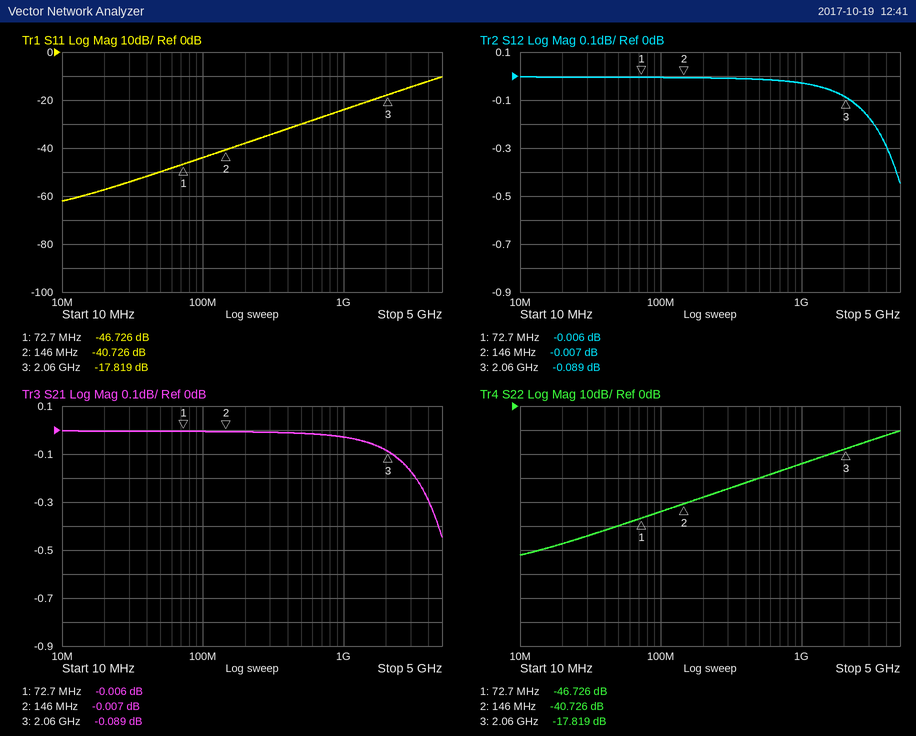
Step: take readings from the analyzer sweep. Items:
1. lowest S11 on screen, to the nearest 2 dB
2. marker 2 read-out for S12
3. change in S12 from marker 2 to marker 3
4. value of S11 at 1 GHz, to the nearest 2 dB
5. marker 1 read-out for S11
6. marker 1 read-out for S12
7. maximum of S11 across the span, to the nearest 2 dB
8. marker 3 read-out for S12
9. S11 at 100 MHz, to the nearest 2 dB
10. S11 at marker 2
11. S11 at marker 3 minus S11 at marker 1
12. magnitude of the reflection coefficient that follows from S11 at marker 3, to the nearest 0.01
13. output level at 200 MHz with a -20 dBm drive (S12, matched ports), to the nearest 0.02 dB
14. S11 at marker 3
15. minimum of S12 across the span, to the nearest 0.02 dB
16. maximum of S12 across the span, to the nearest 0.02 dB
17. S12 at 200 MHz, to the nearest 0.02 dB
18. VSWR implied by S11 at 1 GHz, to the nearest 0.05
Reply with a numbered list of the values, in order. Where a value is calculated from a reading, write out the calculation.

1. -62 dB
2. -0.007 dB
3. -0.089 − (-0.007) = -0.082 dB
4. -24 dB
5. -46.726 dB
6. -0.006 dB
7. -10 dB
8. -0.089 dB
9. -44 dB
10. -40.726 dB
11. -17.819 − (-46.726) = 28.907 dB
12. 10^(-17.819/20) ≈ 0.13
13. -20 dBm + (0.00 dB) = -20.00 dBm
14. -17.819 dB
15. -0.44 dB
16. 0.00 dB
17. 0.00 dB
18. |Γ| = 10^(-24/20) = 0.0631; VSWR = (1 + 0.0631)/(1 − 0.0631) ≈ 1.13, so 1.15 to the nearest 0.05
